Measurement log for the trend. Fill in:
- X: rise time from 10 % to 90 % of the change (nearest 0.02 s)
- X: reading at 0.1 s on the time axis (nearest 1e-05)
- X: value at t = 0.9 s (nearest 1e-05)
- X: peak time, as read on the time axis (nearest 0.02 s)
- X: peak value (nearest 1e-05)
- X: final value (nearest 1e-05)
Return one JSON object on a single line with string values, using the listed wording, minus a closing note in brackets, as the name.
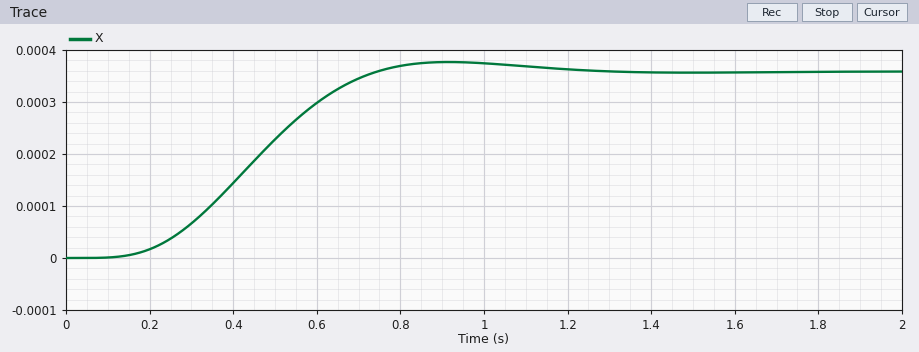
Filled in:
{"X: rise time from 10 % to 90 % of the change": "0.40 s", "X: reading at 0.1 s on the time axis": "0.00000", "X: value at t = 0.9 s": "0.00038", "X: peak time, as read on the time axis": "0.92 s", "X: peak value": "0.00038", "X: final value": "0.00036"}
